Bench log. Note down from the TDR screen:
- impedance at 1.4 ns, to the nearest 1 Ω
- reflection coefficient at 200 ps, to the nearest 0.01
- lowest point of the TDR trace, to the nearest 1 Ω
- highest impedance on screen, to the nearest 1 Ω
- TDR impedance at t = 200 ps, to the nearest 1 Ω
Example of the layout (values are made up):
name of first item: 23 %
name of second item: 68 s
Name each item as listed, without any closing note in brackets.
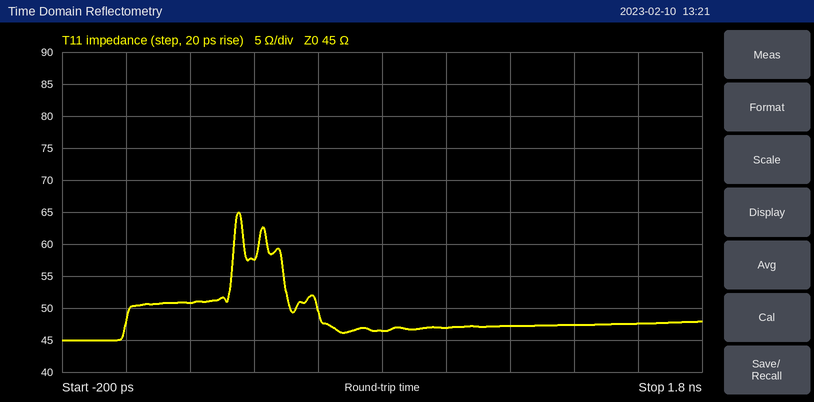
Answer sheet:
impedance at 1.4 ns, to the nearest 1 Ω: 47 Ω
reflection coefficient at 200 ps, to the nearest 0.01: +0.06
lowest point of the TDR trace, to the nearest 1 Ω: 45 Ω
highest impedance on screen, to the nearest 1 Ω: 65 Ω
TDR impedance at t = 200 ps, to the nearest 1 Ω: 51 Ω
